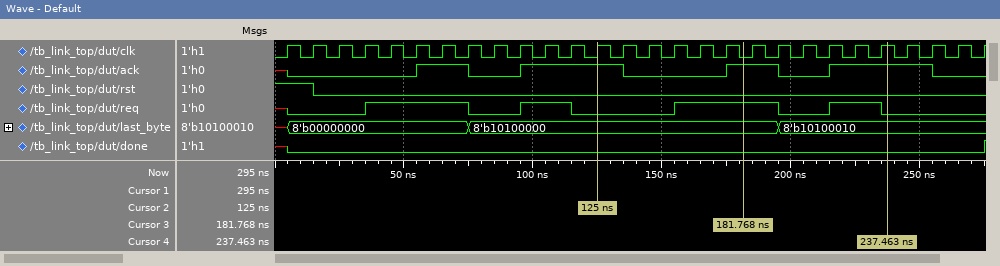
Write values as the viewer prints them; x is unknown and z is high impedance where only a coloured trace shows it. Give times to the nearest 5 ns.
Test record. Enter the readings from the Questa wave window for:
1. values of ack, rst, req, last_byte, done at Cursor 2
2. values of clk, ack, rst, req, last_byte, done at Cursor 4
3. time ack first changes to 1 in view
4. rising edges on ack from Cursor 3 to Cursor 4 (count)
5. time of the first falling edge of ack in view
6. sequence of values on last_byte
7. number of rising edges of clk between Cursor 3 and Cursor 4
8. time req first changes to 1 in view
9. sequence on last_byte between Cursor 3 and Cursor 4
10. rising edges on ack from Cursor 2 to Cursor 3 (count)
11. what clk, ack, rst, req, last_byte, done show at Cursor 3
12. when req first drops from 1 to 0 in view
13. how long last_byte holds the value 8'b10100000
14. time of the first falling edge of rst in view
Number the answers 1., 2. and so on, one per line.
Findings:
1. ack=1, rst=0, req=0, last_byte=8'b10100000, done=0
2. clk=1, ack=1, rst=0, req=0, last_byte=8'b10100010, done=0
3. 55 ns
4. 1
5. 75 ns
6. x, 8'b00000000, 8'b10100000, 8'b10100010
7. 6
8. 35 ns
9. 8'b10100000, 8'b10100010
10. 1
11. clk=0, ack=1, rst=0, req=1, last_byte=8'b10100000, done=0
12. 75 ns
13. 120 ns
14. 15 ns
